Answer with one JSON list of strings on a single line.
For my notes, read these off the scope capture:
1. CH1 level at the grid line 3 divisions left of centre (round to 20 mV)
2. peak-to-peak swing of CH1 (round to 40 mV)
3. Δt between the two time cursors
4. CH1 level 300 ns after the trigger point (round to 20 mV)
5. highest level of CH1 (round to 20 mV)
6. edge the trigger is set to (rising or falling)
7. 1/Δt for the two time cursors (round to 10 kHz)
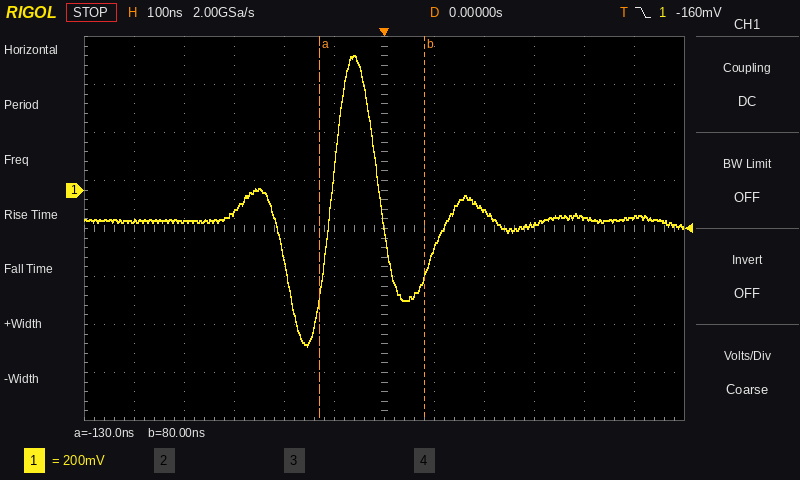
["-100 mV", "1.20 V", "210 ns", "-140 mV", "560 mV", "falling", "4.76 MHz"]
